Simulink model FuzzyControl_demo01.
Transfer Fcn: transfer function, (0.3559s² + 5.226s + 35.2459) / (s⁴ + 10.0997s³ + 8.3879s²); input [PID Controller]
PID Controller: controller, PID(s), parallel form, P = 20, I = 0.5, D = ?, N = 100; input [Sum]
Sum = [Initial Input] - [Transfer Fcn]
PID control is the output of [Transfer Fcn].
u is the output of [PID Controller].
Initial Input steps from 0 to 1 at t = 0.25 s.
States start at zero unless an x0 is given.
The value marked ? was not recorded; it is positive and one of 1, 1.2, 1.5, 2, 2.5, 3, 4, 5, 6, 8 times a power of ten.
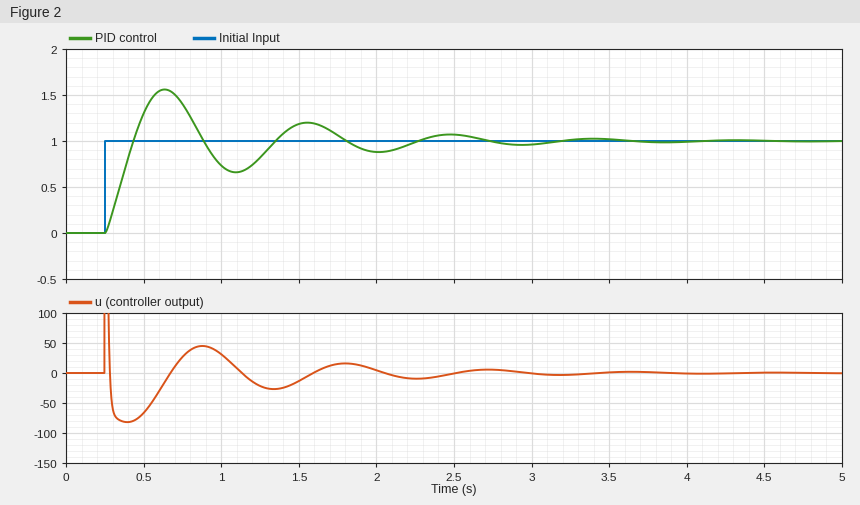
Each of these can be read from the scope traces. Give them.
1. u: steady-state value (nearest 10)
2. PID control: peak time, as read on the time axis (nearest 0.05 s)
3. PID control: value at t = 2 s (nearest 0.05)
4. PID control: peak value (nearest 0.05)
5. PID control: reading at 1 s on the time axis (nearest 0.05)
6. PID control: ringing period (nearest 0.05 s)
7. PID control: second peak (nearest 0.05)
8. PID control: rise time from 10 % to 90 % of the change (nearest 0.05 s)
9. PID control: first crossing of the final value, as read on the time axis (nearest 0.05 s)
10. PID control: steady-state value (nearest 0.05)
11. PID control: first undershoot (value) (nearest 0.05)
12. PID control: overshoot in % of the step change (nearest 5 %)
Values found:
0
0.65 s
0.90
1.55
0.75
0.90 s
1.20
0.15 s
0.45 s
1.00
0.65
55 %
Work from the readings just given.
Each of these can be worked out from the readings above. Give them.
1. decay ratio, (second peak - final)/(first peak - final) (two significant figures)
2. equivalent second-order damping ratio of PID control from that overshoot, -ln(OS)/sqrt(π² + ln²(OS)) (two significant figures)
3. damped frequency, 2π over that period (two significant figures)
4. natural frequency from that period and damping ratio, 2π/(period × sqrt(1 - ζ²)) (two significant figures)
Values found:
0.36
0.19
7.0 rad/s
7.1 rad/s
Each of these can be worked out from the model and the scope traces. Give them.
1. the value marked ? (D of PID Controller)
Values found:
15
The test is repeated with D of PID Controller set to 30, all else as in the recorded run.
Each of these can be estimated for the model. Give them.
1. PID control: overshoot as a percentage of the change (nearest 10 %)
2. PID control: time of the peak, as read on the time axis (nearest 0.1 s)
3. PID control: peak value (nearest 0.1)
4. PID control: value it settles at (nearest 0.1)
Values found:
40 %
0.5 s
1.4
1.0
